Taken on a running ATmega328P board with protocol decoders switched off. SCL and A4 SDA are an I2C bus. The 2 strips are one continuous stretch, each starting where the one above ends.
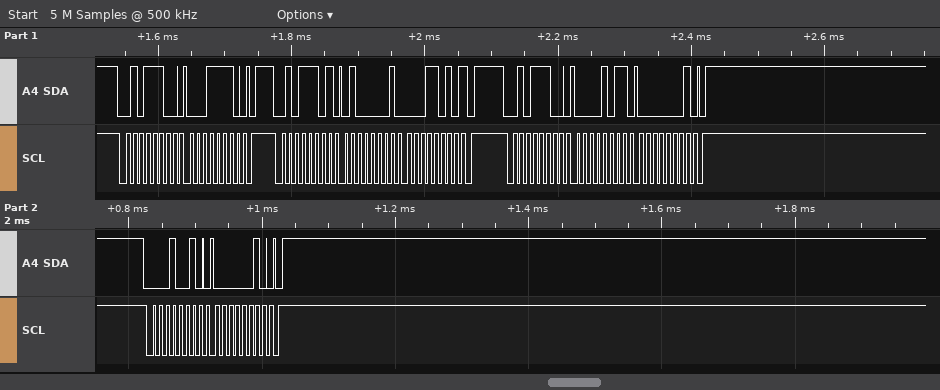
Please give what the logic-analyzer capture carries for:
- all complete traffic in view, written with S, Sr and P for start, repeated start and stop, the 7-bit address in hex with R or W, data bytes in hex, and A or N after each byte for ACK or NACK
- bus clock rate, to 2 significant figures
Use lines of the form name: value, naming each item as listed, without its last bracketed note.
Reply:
all complete traffic in view, written with S, Sr and P for start, repeated start and stop, the 7-bit address in hex with R or W, data bytes in hex, and A or N after each byte for ACK or NACK: S 2EW A 1E A P S 2ER A 41 A 1A N P S 2EW A 0B A 01 A P S 09W A 02 A P
bus clock rate, to 2 significant figures: 100 kHz
